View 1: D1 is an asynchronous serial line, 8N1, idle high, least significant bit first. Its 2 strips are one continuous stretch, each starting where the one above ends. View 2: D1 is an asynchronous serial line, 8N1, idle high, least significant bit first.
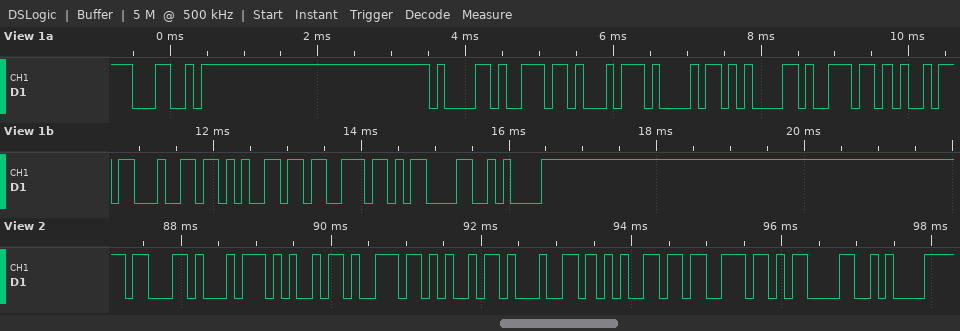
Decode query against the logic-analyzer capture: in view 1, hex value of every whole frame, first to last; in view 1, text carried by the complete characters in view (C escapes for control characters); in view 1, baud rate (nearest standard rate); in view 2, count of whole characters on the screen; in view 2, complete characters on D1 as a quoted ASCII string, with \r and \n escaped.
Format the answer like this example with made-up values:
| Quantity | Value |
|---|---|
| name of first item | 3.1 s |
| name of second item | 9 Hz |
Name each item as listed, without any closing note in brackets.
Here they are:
| Quantity | Value |
|---|---|
| in view 1, hex value of every whole frame, first to last | 4C 61 6E 74 68 61 6E 69 64 65 73 0D 0A |
| in view 1, text carried by the complete characters in view | "Lanthanides\r\n" |
| in view 1, baud rate | 9600 baud |
| in view 2, count of whole characters on the screen | 10 |
| in view 2, complete characters on D1 as a quoted ASCII string, with \r and \n escaped | "ctinides\r\n" |
